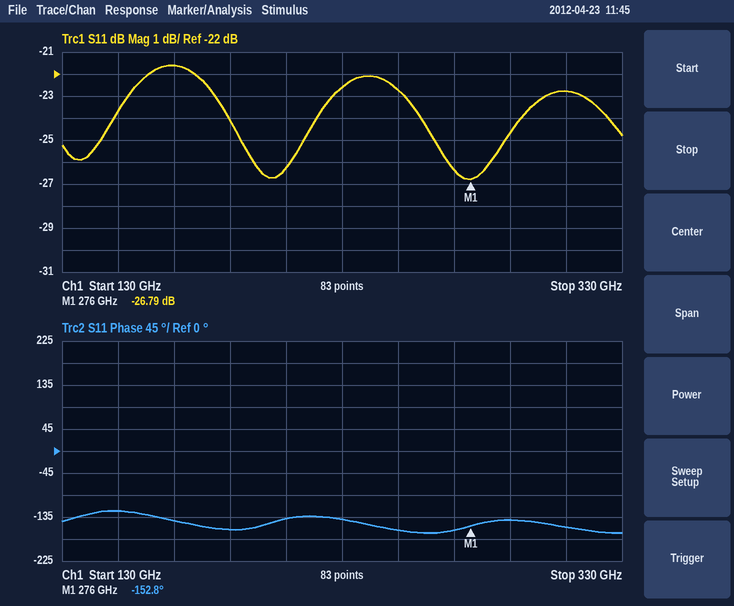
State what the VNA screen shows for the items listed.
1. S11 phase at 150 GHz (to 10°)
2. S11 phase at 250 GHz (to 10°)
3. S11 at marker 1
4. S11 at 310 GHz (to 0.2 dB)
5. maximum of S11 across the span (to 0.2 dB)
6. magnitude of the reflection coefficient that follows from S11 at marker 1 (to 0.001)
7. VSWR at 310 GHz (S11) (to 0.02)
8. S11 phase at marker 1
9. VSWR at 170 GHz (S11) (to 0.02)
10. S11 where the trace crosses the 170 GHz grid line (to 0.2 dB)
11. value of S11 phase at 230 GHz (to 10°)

-120°
-160°
-26.79 dB
-22.8 dB
-21.6 dB
0.046
1.16
-152.8°
1.18
-21.6 dB
-140°
